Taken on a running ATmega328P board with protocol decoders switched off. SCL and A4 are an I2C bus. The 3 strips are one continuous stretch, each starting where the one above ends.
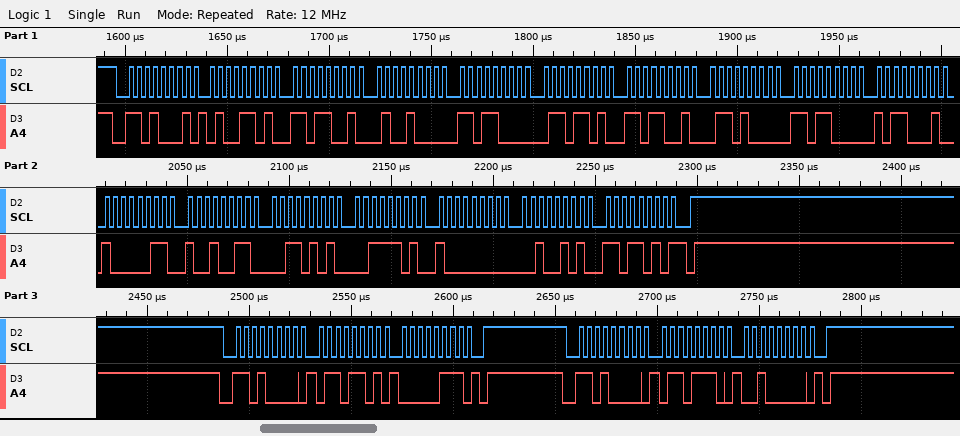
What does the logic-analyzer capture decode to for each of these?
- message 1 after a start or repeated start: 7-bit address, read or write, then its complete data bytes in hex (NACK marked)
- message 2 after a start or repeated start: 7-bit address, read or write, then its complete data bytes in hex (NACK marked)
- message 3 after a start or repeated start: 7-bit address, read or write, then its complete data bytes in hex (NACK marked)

0x68 read: 4D D9 48 D8 6D D9 68 D8 B1 83 93 35 3D 80 25 DA NACK
0x68 write: 6D 07
0x68 write: 6E 20
